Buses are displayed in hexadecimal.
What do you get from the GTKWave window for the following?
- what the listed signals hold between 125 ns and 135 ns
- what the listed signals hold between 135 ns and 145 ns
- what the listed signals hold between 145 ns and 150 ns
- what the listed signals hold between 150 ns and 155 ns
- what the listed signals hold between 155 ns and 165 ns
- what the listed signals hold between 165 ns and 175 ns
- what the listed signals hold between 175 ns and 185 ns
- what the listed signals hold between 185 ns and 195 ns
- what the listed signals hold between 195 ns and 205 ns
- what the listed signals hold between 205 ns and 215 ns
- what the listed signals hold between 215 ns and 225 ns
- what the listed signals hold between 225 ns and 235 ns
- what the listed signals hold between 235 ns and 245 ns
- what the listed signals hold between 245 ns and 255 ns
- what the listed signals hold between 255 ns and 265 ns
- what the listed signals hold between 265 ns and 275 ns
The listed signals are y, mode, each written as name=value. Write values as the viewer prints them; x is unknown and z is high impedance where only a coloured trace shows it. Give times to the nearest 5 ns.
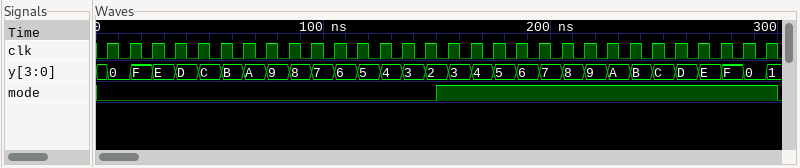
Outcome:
y=4, mode=0
y=3, mode=0
y=2, mode=0
y=2, mode=1
y=3, mode=1
y=4, mode=1
y=5, mode=1
y=6, mode=1
y=7, mode=1
y=8, mode=1
y=9, mode=1
y=A, mode=1
y=B, mode=1
y=C, mode=1
y=D, mode=1
y=E, mode=1
